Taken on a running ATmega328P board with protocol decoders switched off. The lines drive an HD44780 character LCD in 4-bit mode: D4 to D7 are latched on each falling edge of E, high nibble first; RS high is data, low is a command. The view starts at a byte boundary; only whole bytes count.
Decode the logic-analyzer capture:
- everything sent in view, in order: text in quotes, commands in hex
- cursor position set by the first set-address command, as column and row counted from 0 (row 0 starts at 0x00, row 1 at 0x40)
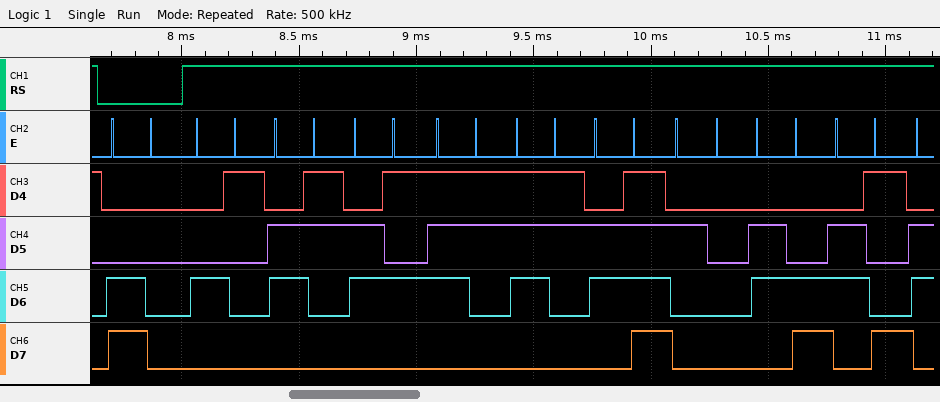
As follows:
0xC0 "Acesso li"
column 0, row 1
